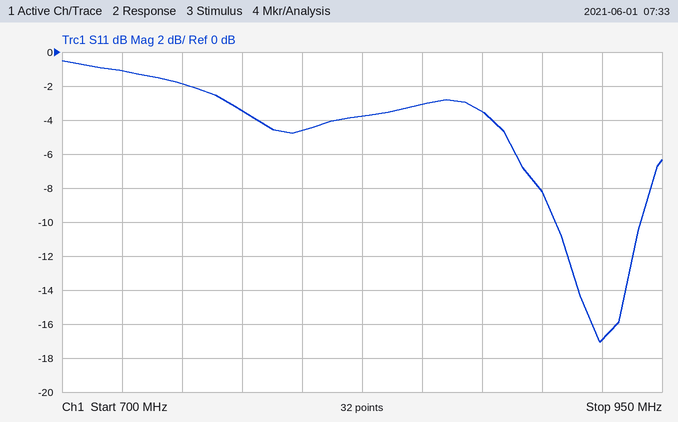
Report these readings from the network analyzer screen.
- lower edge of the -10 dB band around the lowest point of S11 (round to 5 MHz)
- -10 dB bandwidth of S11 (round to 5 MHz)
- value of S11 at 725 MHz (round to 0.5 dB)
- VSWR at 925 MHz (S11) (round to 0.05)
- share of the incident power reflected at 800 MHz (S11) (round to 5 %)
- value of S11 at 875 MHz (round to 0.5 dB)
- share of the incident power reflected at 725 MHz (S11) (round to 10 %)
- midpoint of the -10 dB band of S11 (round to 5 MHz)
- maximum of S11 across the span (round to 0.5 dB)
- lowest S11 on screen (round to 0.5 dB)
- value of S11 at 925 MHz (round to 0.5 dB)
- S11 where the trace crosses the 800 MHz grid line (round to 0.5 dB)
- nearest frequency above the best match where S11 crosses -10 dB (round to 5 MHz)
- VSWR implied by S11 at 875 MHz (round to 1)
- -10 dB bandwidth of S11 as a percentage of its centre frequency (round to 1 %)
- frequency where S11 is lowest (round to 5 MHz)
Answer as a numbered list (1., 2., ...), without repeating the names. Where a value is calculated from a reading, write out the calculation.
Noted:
1. 905 MHz
2. 940 MHz − 905 MHz = 35 MHz
3. -1.0 dB
4. |Γ| = 10^(-17/20) = 0.1413; VSWR = (1 + 0.1413)/(1 − 0.1413) ≈ 1.33, so 1.35 to the nearest 0.05
5. 10^(-4.5/10) ≈ 35 %
6. -3.5 dB
7. 10^(-1/10) ≈ 79.4 %, so 80 % to the nearest 10 %
8. 925 MHz
9. -0.5 dB
10. -17.0 dB
11. -17.0 dB
12. -4.5 dB
13. 940 MHz
14. |Γ| = 10^(-3.5/20) = 0.6683; VSWR = (1 + 0.6683)/(1 − 0.6683) ≈ 5
15. 35 MHz / 922.5 MHz ≈ 4 %
16. 925 MHz
